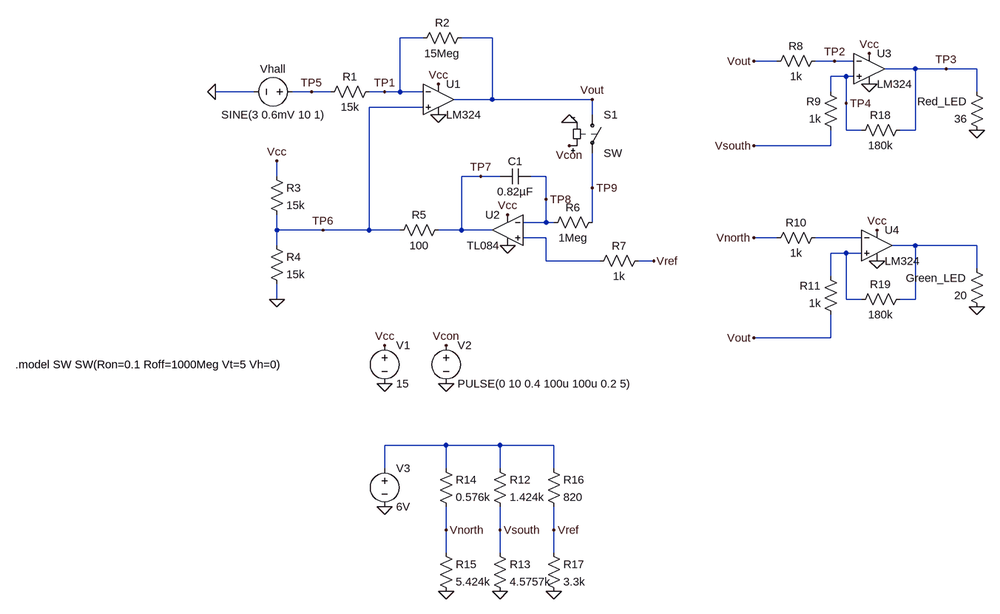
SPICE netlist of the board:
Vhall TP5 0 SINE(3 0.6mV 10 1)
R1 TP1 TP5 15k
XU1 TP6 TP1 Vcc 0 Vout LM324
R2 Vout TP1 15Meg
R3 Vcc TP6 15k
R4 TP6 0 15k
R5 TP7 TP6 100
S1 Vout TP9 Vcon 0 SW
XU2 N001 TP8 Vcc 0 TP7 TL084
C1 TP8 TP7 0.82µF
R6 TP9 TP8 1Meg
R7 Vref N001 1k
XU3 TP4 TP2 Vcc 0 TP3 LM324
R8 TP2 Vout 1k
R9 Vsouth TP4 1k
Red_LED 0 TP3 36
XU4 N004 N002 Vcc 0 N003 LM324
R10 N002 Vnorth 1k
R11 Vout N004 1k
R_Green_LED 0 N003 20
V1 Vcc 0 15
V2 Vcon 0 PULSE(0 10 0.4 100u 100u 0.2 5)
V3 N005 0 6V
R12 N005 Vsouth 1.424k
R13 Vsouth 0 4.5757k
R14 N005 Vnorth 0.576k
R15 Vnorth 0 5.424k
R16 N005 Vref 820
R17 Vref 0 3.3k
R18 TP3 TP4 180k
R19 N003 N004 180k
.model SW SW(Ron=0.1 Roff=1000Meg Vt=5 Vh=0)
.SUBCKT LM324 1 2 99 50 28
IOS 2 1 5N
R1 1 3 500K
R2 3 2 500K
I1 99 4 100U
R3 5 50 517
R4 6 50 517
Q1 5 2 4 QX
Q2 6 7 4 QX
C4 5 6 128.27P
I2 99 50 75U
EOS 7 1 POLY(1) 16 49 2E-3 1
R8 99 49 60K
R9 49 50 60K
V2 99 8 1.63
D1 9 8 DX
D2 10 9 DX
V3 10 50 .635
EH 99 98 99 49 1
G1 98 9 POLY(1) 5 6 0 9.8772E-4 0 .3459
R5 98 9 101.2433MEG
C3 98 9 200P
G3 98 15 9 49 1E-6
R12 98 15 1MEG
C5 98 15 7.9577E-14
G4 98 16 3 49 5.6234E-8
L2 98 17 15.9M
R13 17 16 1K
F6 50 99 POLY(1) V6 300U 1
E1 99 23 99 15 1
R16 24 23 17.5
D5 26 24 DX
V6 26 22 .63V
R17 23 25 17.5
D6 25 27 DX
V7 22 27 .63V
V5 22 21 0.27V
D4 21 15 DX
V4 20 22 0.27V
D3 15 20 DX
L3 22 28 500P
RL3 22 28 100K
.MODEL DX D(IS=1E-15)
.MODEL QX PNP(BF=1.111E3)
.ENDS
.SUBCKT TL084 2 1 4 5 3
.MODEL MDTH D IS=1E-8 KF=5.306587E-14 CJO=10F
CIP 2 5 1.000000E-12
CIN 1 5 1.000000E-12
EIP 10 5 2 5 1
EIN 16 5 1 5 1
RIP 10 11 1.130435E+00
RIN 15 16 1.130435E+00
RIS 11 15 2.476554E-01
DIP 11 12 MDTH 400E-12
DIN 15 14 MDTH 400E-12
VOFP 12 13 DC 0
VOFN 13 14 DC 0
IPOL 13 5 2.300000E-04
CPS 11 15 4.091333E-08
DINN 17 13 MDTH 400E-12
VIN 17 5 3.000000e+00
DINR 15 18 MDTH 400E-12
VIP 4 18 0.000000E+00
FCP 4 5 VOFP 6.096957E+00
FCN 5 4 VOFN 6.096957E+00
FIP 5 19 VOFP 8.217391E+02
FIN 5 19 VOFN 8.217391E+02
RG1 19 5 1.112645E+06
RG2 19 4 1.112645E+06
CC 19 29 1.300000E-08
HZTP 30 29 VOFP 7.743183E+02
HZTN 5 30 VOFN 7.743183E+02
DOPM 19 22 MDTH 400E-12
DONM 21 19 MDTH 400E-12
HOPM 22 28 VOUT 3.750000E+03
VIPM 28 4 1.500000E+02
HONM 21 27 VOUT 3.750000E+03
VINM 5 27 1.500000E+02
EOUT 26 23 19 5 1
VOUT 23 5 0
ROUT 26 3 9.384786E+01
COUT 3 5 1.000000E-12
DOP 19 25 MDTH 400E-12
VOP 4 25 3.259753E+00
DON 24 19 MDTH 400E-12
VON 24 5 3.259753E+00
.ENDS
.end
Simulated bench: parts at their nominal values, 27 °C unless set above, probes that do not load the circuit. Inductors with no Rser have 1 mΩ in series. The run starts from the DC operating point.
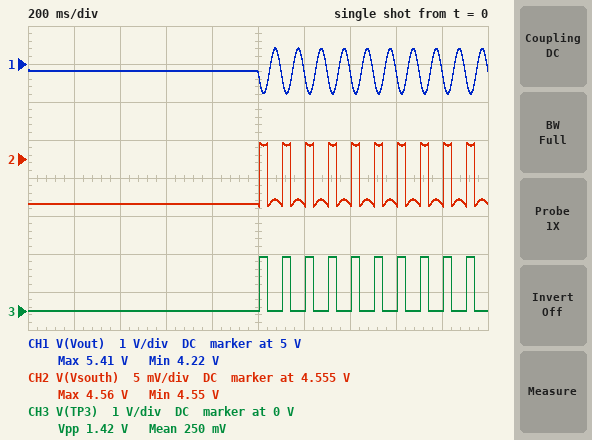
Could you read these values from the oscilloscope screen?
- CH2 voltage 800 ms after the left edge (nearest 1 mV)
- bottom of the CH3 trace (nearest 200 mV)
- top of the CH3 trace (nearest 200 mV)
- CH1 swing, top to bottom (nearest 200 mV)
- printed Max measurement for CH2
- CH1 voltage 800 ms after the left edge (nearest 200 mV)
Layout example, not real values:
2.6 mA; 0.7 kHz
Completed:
4.549 V; 0 V; 1.4 V; 1.2 V; 4.56 V; 4.8 V
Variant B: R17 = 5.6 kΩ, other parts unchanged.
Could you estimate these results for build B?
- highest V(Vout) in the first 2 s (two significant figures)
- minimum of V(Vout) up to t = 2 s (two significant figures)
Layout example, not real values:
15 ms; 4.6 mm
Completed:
5.8 V; 4.6 V
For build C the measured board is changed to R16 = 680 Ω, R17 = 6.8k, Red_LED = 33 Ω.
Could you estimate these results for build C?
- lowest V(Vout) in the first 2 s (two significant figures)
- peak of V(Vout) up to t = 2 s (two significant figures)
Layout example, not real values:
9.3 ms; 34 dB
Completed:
4.9 V; 6.1 V
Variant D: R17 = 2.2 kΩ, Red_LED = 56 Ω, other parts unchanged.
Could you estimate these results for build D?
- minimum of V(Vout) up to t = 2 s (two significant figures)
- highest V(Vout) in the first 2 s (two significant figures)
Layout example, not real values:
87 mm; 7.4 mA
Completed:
3.8 V; 5.0 V
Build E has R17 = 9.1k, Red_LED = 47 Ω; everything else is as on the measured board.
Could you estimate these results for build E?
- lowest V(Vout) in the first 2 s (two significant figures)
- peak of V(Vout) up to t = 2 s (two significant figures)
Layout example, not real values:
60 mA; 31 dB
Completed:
4.9 V; 6.1 V
